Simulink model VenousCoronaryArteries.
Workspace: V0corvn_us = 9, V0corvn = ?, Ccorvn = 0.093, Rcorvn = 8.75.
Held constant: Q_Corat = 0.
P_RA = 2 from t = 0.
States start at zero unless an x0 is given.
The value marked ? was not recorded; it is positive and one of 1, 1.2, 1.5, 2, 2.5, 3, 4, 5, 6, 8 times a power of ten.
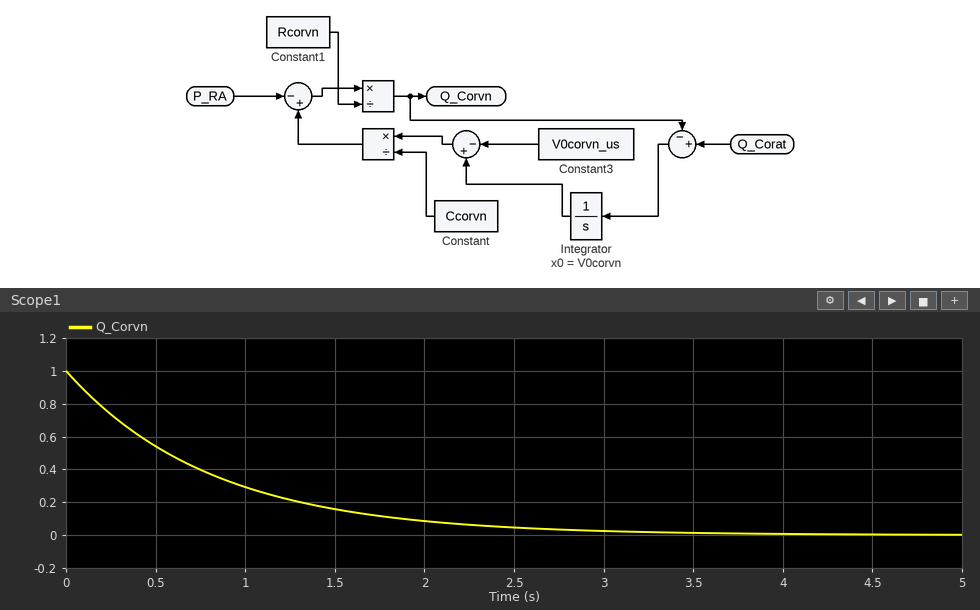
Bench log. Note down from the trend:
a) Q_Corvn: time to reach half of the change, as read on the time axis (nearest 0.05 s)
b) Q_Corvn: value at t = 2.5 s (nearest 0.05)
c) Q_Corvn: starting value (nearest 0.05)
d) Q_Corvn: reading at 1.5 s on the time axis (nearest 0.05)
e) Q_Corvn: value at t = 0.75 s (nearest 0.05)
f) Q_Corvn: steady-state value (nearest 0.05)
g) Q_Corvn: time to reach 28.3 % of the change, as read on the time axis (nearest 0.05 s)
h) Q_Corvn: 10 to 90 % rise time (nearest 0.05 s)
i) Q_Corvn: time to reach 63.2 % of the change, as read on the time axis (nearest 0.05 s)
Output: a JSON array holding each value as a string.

["0.55 s", "0.05", "1.00", "0.15", "0.40", "0.00", "0.25 s", "1.80 s", "0.80 s"]
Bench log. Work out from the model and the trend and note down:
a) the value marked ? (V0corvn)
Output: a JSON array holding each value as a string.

["10"]
